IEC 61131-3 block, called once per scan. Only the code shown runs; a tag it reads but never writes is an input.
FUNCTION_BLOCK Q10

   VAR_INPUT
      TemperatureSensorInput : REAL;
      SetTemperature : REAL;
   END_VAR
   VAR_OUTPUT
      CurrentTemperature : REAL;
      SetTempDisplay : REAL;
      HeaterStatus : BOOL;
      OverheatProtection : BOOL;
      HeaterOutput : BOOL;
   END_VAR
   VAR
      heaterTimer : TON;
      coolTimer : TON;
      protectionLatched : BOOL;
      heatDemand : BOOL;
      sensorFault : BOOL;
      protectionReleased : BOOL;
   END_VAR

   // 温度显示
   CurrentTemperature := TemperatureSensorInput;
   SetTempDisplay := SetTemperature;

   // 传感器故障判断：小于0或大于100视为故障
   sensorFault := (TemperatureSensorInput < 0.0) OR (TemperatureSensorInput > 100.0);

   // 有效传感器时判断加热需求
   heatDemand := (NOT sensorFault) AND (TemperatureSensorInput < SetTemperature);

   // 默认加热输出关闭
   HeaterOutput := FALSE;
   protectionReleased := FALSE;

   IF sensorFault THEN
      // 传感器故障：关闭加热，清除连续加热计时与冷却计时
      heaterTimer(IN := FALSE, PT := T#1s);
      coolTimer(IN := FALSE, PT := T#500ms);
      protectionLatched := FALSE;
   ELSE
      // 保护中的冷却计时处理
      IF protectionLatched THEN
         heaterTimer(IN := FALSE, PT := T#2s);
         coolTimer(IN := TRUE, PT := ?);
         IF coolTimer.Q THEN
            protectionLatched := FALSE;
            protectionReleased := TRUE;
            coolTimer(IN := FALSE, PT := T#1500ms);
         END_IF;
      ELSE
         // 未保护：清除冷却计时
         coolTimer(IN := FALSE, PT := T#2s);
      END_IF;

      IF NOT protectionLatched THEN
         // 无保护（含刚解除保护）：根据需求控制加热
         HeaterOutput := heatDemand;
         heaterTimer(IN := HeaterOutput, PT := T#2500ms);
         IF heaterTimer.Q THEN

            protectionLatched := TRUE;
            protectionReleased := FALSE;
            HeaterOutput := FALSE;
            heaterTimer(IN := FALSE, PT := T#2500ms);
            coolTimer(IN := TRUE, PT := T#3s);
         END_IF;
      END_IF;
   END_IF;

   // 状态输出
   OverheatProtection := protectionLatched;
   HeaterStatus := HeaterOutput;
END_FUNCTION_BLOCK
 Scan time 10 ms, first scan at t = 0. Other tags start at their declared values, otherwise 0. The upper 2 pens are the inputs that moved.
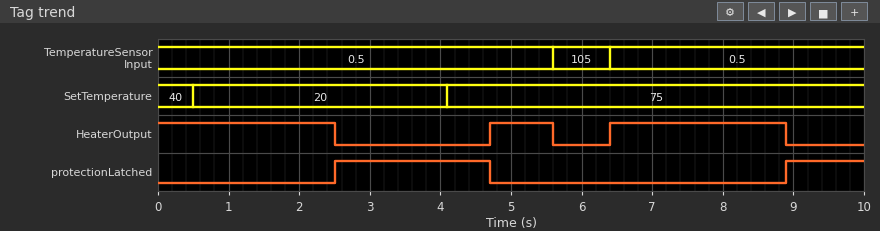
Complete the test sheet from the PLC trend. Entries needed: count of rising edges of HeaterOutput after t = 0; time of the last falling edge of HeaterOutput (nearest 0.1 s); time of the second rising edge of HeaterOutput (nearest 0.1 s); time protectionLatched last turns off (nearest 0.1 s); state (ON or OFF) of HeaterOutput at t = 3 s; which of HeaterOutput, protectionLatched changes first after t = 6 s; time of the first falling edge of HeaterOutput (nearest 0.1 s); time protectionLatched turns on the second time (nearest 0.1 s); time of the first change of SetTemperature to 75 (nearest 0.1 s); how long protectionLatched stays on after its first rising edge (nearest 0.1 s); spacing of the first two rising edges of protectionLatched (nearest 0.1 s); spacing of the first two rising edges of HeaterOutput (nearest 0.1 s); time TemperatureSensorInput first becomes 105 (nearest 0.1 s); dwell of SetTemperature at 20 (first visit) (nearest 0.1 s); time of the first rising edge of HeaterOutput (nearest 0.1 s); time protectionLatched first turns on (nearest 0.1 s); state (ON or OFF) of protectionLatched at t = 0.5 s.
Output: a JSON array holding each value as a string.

["2", "8.9 s", "6.4 s", "4.7 s", "OFF", "HeaterOutput", "2.5 s", "8.9 s", "4.1 s", "2.2 s", "6.4 s", "1.7 s", "5.6 s", "3.6 s", "4.7 s", "2.5 s", "OFF"]
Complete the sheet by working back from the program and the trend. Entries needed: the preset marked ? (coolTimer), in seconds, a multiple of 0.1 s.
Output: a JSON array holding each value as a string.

["2.2 s"]
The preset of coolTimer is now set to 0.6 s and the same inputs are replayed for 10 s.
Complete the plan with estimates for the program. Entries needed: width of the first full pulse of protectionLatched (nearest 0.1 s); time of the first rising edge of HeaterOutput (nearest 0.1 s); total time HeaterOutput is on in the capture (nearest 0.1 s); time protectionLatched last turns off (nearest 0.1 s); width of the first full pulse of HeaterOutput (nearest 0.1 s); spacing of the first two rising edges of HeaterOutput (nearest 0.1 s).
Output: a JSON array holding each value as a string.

["0.6 s", "3.1 s", "8.0 s", "9.5 s", "2.5 s", "3.3 s"]
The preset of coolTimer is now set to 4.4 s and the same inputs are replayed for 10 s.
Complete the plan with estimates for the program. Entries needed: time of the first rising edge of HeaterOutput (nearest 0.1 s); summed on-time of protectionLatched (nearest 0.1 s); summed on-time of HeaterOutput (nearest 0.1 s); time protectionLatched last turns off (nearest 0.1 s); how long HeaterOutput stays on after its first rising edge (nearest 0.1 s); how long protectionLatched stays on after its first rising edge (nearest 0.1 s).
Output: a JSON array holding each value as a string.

["6.4 s", "4.2 s", "5.0 s", "5.6 s", "2.5 s", "3.1 s"]
